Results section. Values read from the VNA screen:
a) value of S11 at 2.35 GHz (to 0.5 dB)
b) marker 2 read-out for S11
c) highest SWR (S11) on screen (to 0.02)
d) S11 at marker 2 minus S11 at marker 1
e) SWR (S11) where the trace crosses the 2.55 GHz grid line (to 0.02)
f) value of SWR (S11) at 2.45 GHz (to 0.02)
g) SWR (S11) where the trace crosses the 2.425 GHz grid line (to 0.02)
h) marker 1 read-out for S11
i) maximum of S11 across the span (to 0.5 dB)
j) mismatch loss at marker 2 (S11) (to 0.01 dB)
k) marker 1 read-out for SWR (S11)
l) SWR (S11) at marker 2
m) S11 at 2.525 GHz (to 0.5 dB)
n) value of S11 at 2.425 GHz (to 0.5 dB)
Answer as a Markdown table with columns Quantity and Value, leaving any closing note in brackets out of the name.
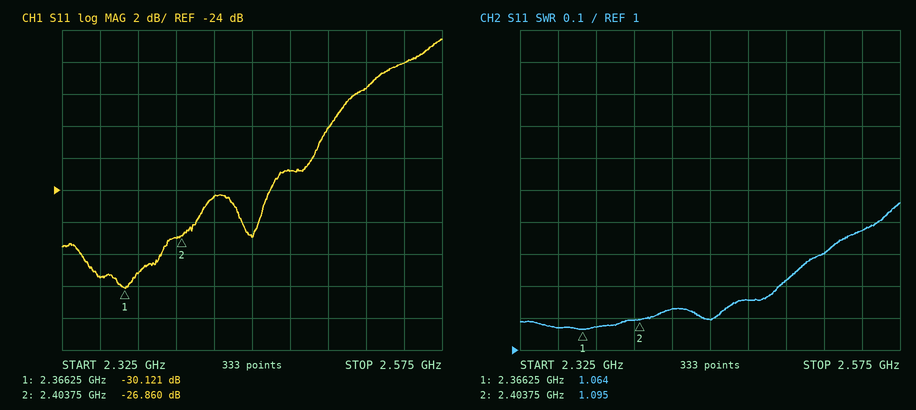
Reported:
| Quantity | Value |
|---|---|
| value of S11 at 2.35 GHz | -29.5 dB |
| marker 2 read-out for S11 | -26.860 dB |
| highest SWR (S11) on screen | 1.46 |
| S11 at marker 2 minus S11 at marker 1 | 3.261 dB |
| SWR (S11) where the trace crosses the 2.55 GHz grid line | 1.38 |
| value of SWR (S11) at 2.45 GHz | 1.10 |
| SWR (S11) where the trace crosses the 2.425 GHz grid line | 1.12 |
| marker 1 read-out for S11 | -30.121 dB |
| maximum of S11 across the span | -14.5 dB |
| mismatch loss at marker 2 (S11) | 0.01 dB |
| marker 1 read-out for SWR | 1.064 |
| SWR (S11) at marker 2 | 1.095 |
| S11 at 2.525 GHz | -17.5 dB |
| value of S11 at 2.425 GHz | -24.5 dB |
